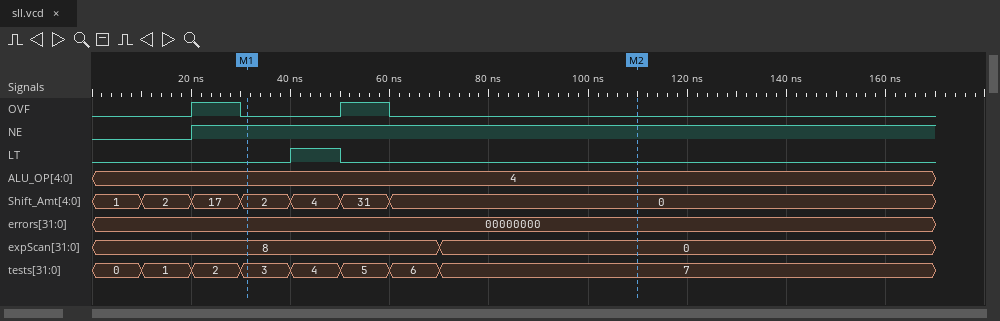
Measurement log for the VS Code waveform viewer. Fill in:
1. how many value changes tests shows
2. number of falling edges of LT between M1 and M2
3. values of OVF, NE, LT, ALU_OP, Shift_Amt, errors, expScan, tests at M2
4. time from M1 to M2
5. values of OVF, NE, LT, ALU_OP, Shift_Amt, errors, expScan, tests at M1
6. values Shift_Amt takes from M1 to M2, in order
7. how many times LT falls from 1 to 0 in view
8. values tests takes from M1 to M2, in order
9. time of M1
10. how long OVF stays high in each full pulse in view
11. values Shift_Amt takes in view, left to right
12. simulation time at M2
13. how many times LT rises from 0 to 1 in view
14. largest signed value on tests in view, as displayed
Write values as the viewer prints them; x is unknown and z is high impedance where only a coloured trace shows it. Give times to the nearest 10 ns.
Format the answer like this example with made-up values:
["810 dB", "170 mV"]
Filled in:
["7", "1", "OVF=0, NE=1, LT=0, ALU_OP=4, Shift_Amt=0, errors=00000000, expScan=0, tests=7", "80 ns", "OVF=0, NE=1, LT=0, ALU_OP=4, Shift_Amt=2, errors=00000000, expScan=8, tests=3", "2, 4, 31, 0", "1", "3, 4, 5, 6, 7", "30 ns", "10 ns, 10 ns", "1, 2, 17, 2, 4, 31, 0", "110 ns", "1", "7"]
